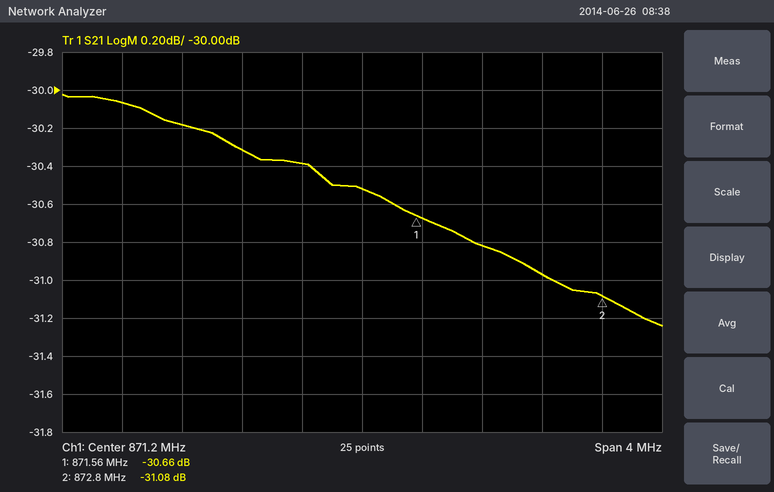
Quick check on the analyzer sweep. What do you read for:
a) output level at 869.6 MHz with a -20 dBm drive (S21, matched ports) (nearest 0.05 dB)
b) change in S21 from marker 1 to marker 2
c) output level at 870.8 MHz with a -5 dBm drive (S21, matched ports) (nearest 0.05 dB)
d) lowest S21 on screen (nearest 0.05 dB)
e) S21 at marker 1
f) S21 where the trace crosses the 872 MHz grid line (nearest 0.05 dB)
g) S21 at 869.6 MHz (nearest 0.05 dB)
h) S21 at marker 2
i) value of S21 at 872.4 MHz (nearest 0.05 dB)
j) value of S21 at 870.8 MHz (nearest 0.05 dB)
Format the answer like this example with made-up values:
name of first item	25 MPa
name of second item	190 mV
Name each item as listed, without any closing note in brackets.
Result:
output level at 869.6 MHz with a -20 dBm drive (S21, matched ports)	-50.05 dBm
change in S21 from marker 1 to marker 2	-0.42 dB
output level at 870.8 MHz with a -5 dBm drive (S21, matched ports)	-35.40 dBm
lowest S21 on screen	-31.25 dB
S21 at marker 1	-30.66 dB
S21 where the trace crosses the 872 MHz grid line	-30.80 dB
S21 at 869.6 MHz	-30.05 dB
S21 at marker 2	-31.08 dB
value of S21 at 872.4 MHz	-30.95 dB
value of S21 at 870.8 MHz	-30.40 dB
